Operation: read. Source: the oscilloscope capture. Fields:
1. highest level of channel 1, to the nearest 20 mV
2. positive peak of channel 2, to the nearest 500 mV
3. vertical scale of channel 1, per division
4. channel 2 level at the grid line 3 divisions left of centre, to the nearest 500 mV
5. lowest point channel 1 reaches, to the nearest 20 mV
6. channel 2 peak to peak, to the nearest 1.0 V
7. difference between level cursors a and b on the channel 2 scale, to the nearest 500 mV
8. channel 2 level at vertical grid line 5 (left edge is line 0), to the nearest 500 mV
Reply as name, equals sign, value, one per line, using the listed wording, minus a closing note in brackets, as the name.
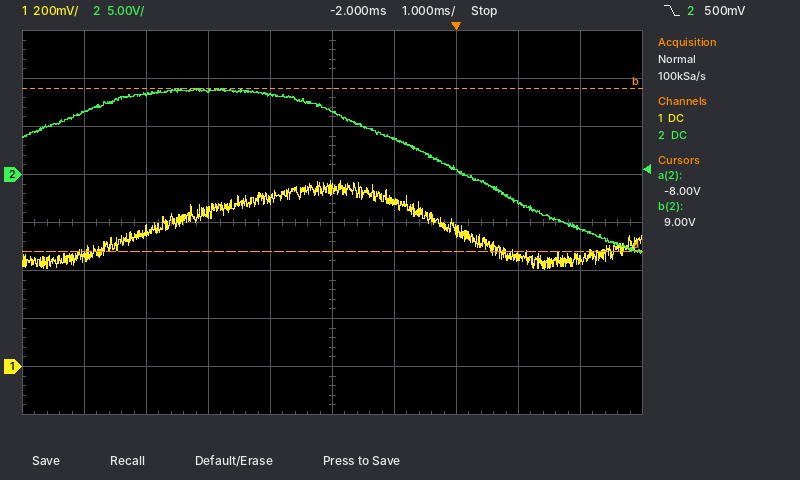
highest level of channel 1, to the nearest 20 mV = 780 mV
positive peak of channel 2, to the nearest 500 mV = 9.0 V
vertical scale of channel 1, per division = 200 mV
channel 2 level at the grid line 3 divisions left of centre, to the nearest 500 mV = 8.5 V
lowest point channel 1 reaches, to the nearest 20 mV = 400 mV
channel 2 peak to peak, to the nearest 1.0 V = 17.0 V
difference between level cursors a and b on the channel 2 scale, to the nearest 500 mV = 17.0 V
channel 2 level at vertical grid line 5 (left edge is line 0), to the nearest 500 mV = 6.5 V
